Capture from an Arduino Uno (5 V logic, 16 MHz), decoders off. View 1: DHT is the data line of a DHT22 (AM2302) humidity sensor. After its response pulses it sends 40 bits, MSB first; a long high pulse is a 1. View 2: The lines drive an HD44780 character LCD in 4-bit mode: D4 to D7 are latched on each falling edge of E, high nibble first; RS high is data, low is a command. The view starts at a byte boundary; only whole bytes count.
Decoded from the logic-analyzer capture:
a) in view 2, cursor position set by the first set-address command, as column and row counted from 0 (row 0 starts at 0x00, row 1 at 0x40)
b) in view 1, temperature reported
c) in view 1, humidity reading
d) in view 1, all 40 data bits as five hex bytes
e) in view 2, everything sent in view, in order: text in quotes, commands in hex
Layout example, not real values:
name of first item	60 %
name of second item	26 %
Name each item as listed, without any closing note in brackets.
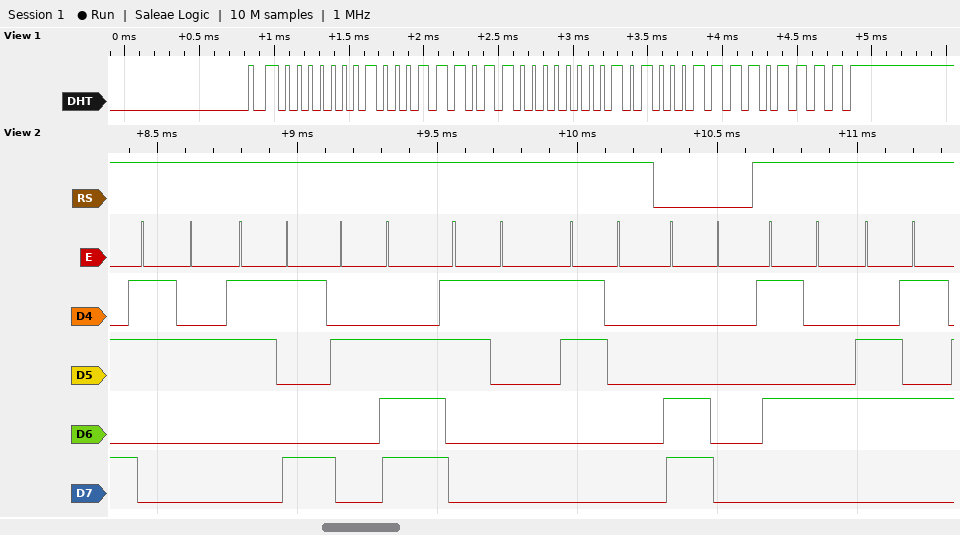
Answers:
in view 2, cursor position set by the first set-address command, as column and row counted from 0	column 0, row 1
in view 1, temperature reported	-8.1 °C
in view 1, humidity reading	28.5 %
in view 1, all 40 data bits as five hex bytes	01 1D 80 51 EF
in view 2, everything sent in view, in order: text in quotes, commands in hex	"29.10" 0xC0 "Te"
